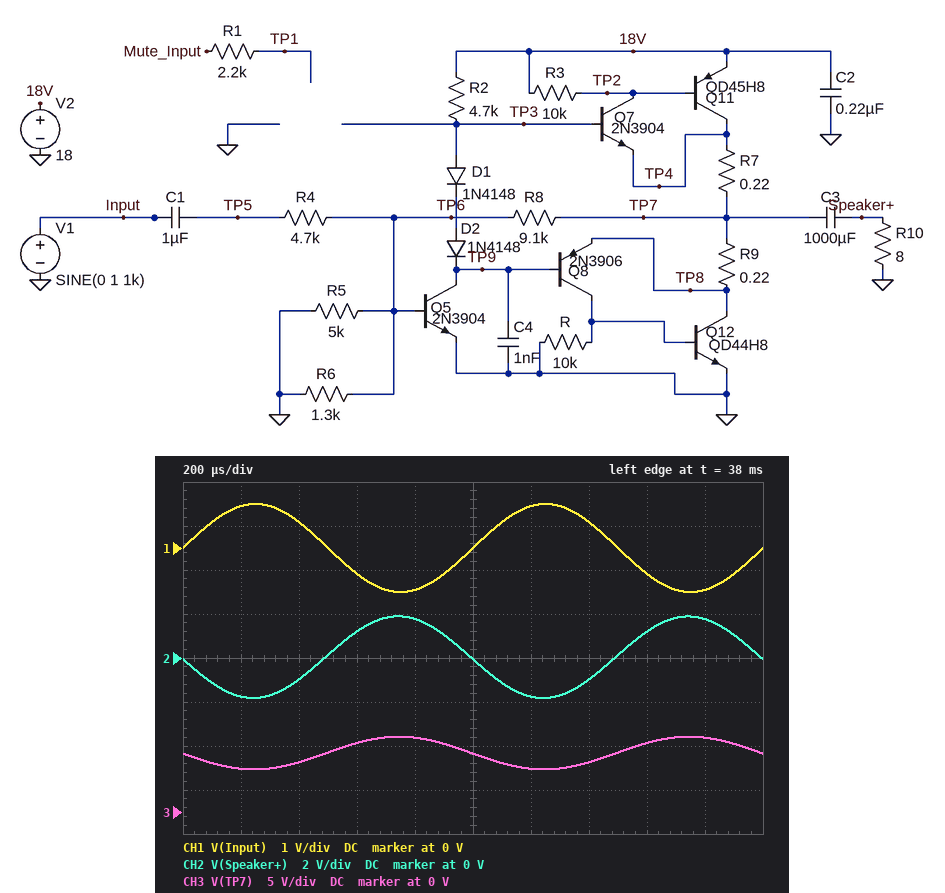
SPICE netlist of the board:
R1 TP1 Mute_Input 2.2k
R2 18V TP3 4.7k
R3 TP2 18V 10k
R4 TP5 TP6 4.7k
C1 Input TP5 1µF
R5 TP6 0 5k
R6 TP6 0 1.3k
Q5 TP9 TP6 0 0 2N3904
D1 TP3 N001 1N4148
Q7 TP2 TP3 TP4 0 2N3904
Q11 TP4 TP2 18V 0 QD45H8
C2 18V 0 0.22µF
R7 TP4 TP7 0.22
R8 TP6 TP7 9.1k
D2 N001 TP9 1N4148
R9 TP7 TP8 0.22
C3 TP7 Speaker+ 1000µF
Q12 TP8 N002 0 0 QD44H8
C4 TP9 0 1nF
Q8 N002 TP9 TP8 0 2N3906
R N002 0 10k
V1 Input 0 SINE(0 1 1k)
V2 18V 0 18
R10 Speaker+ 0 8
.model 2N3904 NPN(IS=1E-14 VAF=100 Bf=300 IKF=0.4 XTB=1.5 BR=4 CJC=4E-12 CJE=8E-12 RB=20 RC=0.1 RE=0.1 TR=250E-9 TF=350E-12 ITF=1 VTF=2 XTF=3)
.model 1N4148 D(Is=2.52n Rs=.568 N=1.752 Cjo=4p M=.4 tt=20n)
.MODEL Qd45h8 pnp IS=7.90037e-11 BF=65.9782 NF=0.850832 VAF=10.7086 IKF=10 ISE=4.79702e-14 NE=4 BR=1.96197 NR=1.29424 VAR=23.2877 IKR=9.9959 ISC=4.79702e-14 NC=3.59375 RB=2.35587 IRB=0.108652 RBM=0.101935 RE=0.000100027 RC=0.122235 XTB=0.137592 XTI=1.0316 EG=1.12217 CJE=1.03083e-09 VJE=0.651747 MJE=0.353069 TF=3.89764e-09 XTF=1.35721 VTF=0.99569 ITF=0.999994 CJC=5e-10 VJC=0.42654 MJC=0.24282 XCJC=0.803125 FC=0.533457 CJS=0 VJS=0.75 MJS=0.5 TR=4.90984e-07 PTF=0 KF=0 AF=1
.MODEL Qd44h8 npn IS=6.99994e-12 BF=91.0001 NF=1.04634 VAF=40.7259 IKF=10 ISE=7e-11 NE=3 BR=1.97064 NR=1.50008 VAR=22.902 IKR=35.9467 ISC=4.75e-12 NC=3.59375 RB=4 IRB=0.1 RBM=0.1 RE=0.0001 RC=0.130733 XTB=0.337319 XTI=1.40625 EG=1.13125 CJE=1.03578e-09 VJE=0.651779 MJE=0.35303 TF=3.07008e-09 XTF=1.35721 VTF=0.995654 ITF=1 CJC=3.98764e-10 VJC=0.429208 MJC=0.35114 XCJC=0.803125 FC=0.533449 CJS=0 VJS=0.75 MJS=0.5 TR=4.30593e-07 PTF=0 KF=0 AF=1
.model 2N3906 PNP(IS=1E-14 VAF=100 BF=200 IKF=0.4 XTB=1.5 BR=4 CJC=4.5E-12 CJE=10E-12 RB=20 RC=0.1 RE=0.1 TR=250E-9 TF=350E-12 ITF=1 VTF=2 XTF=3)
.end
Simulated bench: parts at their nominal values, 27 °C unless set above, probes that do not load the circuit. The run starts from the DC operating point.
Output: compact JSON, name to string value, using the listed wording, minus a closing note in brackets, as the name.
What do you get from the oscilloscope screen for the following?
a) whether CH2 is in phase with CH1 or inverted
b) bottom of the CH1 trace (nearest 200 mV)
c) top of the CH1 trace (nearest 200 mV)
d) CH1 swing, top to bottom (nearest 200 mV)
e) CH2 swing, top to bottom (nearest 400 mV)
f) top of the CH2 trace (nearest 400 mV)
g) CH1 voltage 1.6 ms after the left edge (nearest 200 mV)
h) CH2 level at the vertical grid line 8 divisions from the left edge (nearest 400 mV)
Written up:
{"whether CH2 is in phase with CH1 or inverted": "inverted", "bottom of the CH1 trace": "-1.0 V", "top of the CH1 trace": "1.0 V", "CH1 swing, top to bottom": "2.0 V", "CH2 swing, top to bottom": "3.6 V", "top of the CH2 trace": "2.0 V", "CH1 voltage 1.6 ms after the left edge": "-600 mV", "CH2 level at the vertical grid line 8 divisions from the left edge": "1.2 V"}
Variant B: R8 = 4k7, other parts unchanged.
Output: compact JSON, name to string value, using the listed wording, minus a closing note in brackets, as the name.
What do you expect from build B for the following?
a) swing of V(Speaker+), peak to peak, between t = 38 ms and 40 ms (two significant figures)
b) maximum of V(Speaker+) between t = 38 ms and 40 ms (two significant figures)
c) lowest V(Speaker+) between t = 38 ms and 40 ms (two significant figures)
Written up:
{"swing of V(Speaker+), peak to peak, between t = 38 ms and 40 ms": "2.0 V", "maximum of V(Speaker+) between t = 38 ms and 40 ms": "1.0 V", "lowest V(Speaker+) between t = 38 ms and 40 ms": "-960 mV"}
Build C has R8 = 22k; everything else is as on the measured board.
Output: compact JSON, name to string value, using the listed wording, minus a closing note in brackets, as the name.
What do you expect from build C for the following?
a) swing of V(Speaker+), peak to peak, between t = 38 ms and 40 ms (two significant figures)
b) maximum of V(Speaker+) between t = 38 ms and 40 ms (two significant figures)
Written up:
{"swing of V(Speaker+), peak to peak, between t = 38 ms and 40 ms": "6.5 V", "maximum of V(Speaker+) between t = 38 ms and 40 ms": "3.0 V"}
